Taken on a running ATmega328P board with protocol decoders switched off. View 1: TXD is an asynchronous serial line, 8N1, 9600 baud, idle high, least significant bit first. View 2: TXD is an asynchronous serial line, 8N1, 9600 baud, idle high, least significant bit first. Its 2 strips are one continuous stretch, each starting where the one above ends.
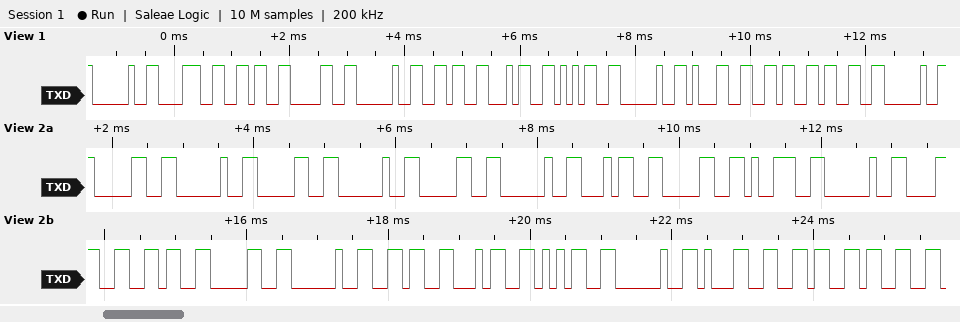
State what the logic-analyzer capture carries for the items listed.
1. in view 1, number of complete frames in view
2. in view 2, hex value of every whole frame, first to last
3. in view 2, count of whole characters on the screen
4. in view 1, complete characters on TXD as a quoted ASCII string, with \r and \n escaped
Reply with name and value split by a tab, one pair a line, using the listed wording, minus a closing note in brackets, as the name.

in view 1, number of complete frames in view	13
in view 2, hex value of every whole frame, first to last	30 20 30 20 30 20 34 30 39 20 38 36 30 20 36 34 35 20 31 36 33
in view 2, count of whole characters on the screen	21
in view 1, complete characters on TXD as a quoted ASCII string, with \r and \n escaped	" 860 645 163 "
